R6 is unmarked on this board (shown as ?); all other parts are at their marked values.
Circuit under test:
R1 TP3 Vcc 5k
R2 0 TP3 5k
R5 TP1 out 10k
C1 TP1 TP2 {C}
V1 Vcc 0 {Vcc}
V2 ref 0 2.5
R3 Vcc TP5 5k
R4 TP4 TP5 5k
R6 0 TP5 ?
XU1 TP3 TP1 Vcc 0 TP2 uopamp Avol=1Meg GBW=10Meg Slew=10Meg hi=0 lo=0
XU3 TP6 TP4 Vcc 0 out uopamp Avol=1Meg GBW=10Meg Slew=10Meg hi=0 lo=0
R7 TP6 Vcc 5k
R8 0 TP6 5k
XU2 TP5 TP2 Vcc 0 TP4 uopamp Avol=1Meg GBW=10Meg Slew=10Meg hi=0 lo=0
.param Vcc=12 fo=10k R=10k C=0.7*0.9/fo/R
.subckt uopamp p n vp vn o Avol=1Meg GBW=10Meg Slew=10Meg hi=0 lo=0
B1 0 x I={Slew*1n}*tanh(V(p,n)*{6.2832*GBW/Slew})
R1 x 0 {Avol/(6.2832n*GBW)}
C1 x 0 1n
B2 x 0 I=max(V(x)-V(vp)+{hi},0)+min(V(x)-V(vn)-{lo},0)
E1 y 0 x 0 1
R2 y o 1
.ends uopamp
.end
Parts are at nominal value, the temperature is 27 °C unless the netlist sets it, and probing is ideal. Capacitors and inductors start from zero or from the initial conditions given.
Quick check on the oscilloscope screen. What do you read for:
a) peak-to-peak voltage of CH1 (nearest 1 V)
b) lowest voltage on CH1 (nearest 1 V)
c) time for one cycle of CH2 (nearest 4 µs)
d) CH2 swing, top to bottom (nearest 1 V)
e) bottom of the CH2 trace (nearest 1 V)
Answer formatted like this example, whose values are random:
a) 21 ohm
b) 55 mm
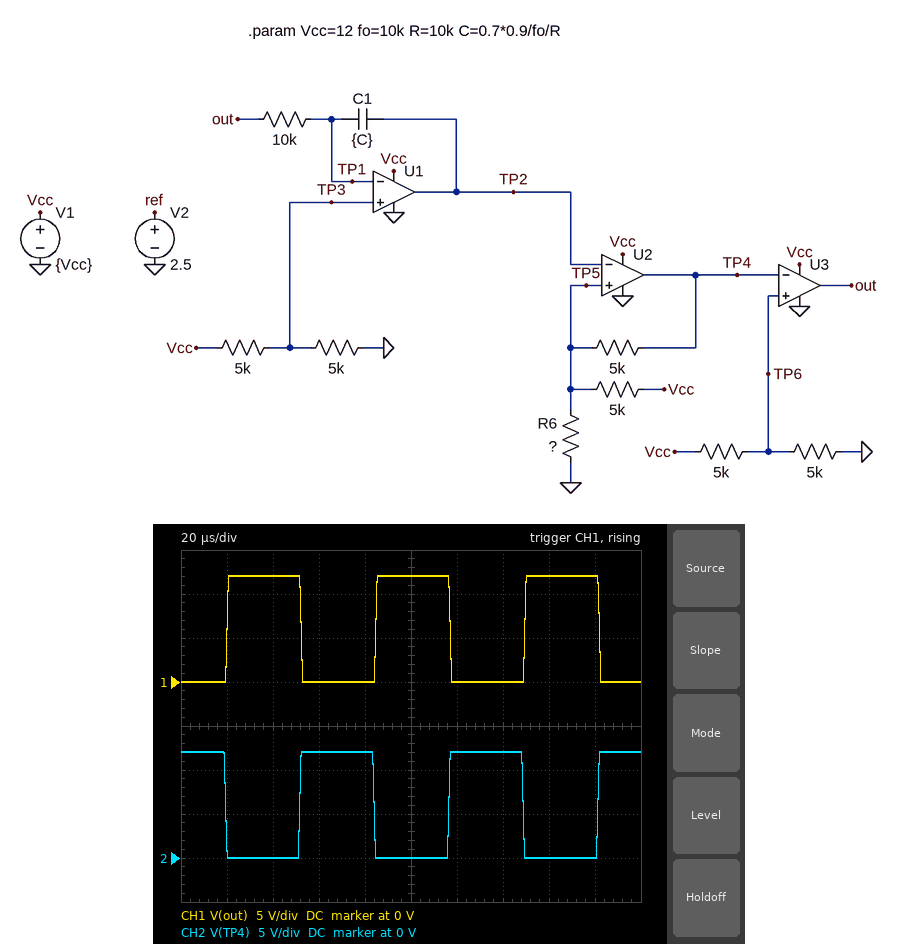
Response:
a) 12 V
b) 0 V
c) 64 µs
d) 12 V
e) 0 V
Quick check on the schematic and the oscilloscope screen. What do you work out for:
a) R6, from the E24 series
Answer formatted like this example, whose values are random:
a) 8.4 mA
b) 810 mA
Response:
a) 2.2 kΩ
